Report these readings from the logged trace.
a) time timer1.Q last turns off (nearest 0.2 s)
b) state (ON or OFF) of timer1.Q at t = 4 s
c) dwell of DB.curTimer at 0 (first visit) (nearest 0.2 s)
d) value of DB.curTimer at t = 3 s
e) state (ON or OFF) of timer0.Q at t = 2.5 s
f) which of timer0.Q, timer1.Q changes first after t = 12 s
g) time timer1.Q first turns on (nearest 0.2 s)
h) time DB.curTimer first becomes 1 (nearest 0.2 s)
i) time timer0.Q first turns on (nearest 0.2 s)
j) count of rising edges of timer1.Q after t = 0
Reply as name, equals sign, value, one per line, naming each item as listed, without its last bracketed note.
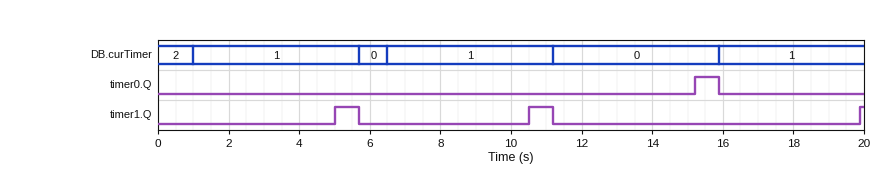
time timer1.Q last turns off = 11.2 s
state (ON or OFF) of timer1.Q at t = 4 s = OFF
dwell of DB.curTimer at 0 (first visit) = 0.8 s
value of DB.curTimer at t = 3 s = 1
state (ON or OFF) of timer0.Q at t = 2.5 s = OFF
which of timer0.Q, timer1.Q changes first after t = 12 s = timer0.Q
time timer1.Q first turns on = 5.0 s
time DB.curTimer first becomes 1 = 1.0 s
time timer0.Q first turns on = 15.2 s
count of rising edges of timer1.Q after t = 0 = 3
